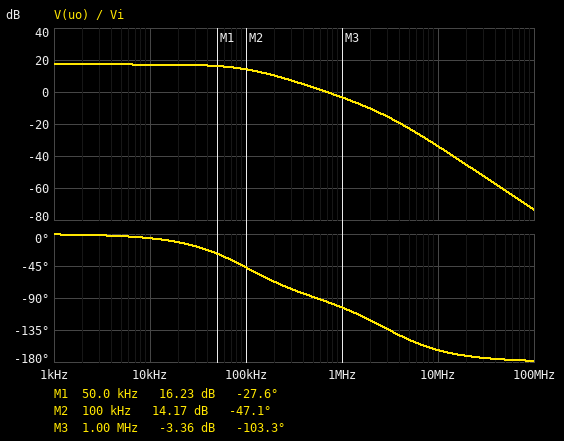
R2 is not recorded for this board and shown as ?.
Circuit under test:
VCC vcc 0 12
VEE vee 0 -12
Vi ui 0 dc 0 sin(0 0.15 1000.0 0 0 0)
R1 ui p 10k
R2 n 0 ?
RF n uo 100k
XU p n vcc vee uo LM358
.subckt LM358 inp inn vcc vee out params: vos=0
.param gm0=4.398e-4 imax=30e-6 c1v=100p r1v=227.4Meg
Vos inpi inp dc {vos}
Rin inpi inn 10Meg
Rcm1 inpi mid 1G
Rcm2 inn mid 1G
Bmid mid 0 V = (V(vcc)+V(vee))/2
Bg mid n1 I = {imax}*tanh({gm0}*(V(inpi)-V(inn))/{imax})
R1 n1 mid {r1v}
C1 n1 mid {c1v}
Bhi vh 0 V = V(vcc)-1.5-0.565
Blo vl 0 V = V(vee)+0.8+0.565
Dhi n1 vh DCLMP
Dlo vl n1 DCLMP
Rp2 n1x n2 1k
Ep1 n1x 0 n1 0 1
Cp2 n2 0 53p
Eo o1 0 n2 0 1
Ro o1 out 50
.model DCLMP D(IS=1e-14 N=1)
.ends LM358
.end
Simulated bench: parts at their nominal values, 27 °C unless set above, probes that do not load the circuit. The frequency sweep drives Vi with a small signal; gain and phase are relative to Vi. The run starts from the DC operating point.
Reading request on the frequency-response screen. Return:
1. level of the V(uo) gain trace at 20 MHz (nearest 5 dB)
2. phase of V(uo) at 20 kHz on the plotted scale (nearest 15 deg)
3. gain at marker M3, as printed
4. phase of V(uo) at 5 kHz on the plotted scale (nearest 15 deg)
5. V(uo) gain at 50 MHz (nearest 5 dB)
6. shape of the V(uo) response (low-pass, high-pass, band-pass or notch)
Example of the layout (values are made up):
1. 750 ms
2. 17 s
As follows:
1. -45 dB
2. -15 deg
3. -3.36 dB
4. 0 deg
5. -60 dB
6. low-pass
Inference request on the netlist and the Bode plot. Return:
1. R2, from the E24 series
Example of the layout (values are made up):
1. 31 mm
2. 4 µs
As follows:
1. 16 kΩ
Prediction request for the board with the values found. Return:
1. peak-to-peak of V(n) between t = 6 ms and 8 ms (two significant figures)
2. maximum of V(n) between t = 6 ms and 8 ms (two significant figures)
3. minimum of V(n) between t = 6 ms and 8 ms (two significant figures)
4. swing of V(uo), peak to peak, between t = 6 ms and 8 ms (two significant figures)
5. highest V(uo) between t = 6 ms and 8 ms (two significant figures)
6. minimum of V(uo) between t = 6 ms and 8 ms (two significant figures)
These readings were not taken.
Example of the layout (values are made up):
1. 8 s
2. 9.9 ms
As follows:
1. 300 mV
2. 150 mV
3. -150 mV
4. 2.2 V
5. 1.1 V
6. -1.1 V
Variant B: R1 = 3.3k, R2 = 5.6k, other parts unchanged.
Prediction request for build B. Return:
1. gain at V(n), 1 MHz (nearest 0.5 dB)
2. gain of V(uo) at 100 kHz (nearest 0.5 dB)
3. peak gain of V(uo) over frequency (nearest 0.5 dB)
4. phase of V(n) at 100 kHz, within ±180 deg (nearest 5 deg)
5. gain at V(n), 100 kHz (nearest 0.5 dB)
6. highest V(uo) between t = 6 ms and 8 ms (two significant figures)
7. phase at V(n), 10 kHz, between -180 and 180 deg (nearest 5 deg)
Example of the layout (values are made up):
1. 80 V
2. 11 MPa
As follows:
1. -29.0 dB
2. 16.5 dB
3. 25.5 dB
4. -70 deg
5. -9.0 dB
6. 2.8 V
7. -15 deg
